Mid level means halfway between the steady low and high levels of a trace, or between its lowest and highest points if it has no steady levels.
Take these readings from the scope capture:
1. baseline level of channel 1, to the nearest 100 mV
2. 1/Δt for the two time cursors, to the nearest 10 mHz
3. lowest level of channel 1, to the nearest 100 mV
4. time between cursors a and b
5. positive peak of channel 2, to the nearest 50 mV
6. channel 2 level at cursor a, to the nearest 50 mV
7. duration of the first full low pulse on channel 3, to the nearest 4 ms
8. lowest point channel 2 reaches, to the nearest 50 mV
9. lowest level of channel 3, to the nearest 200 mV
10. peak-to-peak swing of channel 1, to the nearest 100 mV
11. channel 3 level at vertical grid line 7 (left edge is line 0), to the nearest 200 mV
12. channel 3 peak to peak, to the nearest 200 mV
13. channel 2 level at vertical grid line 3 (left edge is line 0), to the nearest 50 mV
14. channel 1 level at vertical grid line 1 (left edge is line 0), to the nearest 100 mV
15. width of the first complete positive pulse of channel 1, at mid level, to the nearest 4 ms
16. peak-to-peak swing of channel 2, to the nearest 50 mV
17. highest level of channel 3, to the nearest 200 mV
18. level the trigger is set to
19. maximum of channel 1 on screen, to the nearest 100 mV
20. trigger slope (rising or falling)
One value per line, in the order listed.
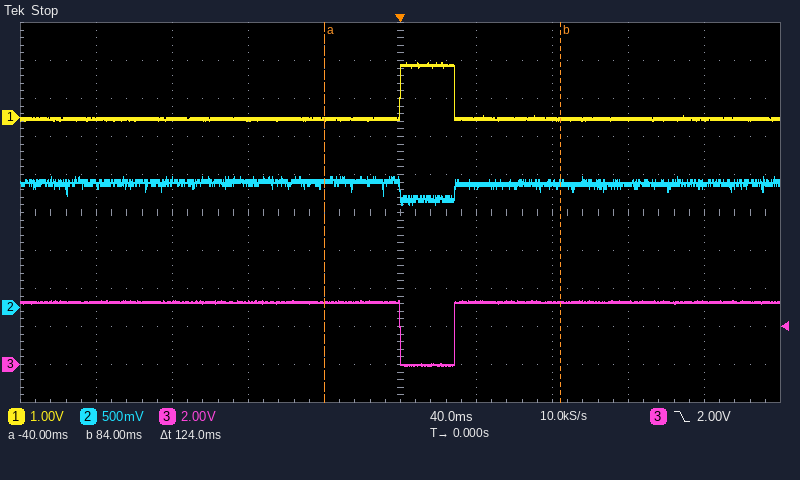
0.0 V
8.06 Hz
-100 mV
124 ms
1.70 V
1.65 V
28 ms
1.35 V
0.0 V
1.5 V
3.2 V
3.4 V
1.65 V
0.0 V
28 ms
350 mV
3.4 V
2.00 V
1.4 V
falling
